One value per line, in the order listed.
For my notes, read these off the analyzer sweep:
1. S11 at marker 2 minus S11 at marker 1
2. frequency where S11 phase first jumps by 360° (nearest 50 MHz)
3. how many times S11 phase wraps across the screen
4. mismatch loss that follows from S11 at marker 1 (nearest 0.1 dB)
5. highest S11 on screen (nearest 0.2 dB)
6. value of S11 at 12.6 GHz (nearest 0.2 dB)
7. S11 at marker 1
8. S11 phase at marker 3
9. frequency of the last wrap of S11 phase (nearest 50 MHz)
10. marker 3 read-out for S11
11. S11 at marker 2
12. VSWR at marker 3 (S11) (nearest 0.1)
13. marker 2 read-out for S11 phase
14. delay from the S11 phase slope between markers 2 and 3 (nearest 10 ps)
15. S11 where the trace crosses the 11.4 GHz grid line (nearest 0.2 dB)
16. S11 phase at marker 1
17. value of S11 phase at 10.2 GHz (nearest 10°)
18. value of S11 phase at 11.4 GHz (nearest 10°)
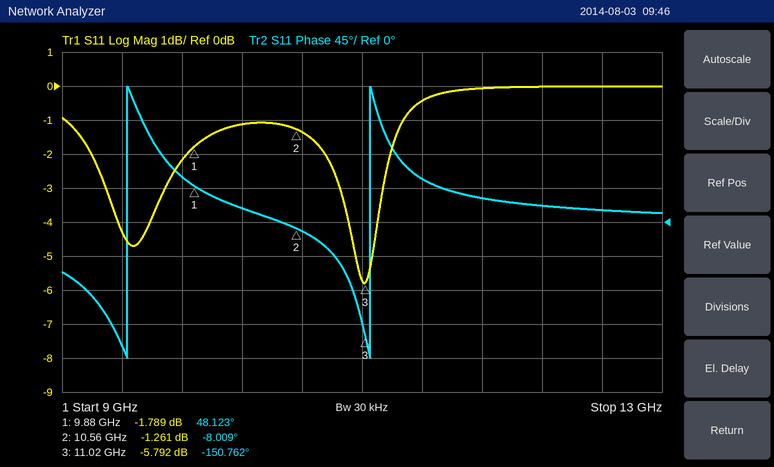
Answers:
0.528 dB
9.45 GHz
2
4.7 dB
0.0 dB
0.0 dB
-1.789 dB
-150.762°
11.05 GHz
-5.792 dB
-1.261 dB
3.1
-8.009°
860 ps
-0.4 dB
48.123°
20°
60°
